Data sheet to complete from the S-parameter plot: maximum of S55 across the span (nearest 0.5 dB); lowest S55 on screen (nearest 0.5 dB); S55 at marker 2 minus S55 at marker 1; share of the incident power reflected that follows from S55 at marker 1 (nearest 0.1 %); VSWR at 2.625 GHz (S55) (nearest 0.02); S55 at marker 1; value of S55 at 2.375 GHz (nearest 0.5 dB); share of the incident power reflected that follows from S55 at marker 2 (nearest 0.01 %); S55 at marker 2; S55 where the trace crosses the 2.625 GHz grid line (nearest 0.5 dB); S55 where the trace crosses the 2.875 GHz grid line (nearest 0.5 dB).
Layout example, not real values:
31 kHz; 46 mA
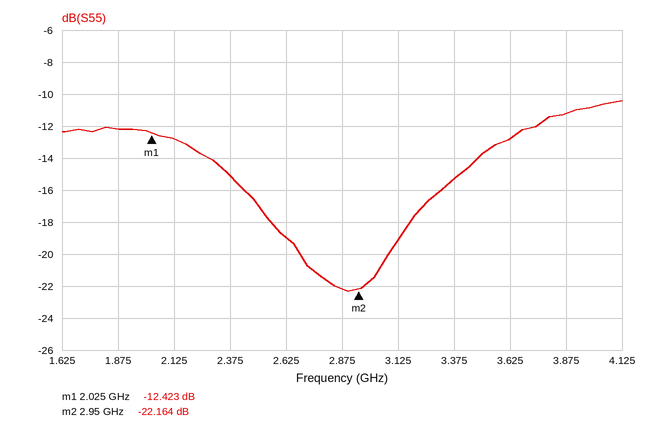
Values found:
-10.5 dB; -22.5 dB; -9.741 dB; 5.7 %; 1.26; -12.423 dB; -15.0 dB; 0.61 %; -22.164 dB; -19.0 dB; -22.0 dB
